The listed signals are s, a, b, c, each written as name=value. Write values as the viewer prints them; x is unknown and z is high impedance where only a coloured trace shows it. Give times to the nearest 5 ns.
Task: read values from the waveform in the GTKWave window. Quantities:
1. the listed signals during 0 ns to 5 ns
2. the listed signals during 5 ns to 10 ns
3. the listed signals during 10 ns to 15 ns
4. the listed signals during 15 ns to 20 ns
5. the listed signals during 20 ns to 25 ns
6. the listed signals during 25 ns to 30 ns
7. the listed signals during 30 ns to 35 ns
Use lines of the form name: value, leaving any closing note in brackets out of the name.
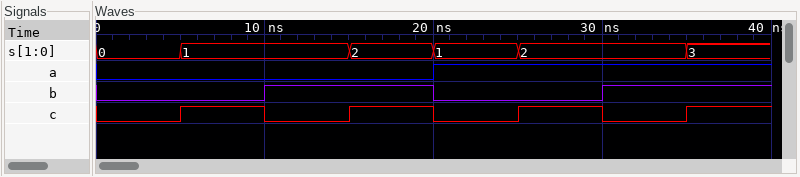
the listed signals during 0 ns to 5 ns: s=0, a=0, b=0, c=0
the listed signals during 5 ns to 10 ns: s=1, a=0, b=0, c=1
the listed signals during 10 ns to 15 ns: s=1, a=0, b=1, c=0
the listed signals during 15 ns to 20 ns: s=2, a=0, b=1, c=1
the listed signals during 20 ns to 25 ns: s=1, a=1, b=0, c=0
the listed signals during 25 ns to 30 ns: s=2, a=1, b=0, c=1
the listed signals during 30 ns to 35 ns: s=2, a=1, b=1, c=0
